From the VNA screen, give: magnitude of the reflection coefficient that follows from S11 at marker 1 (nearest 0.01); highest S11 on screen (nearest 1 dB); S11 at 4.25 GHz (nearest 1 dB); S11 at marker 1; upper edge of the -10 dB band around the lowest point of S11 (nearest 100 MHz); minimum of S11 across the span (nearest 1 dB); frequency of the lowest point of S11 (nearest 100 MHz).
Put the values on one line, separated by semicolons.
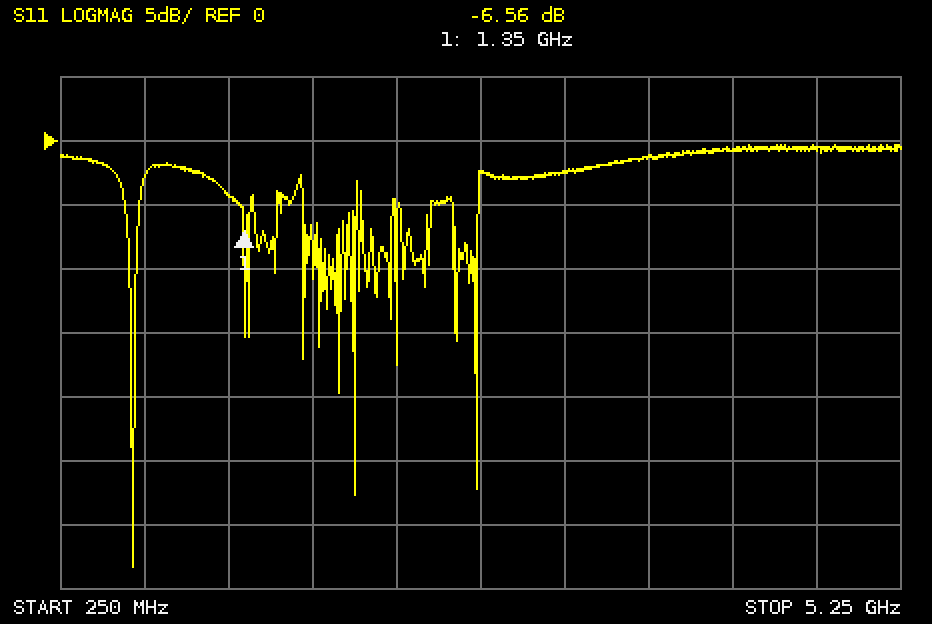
0.47; 0 dB; -1 dB; -6.56 dB; 700 MHz; -33 dB; 700 MHz
